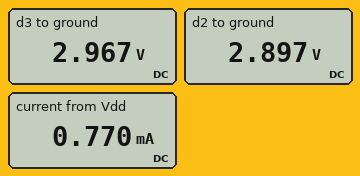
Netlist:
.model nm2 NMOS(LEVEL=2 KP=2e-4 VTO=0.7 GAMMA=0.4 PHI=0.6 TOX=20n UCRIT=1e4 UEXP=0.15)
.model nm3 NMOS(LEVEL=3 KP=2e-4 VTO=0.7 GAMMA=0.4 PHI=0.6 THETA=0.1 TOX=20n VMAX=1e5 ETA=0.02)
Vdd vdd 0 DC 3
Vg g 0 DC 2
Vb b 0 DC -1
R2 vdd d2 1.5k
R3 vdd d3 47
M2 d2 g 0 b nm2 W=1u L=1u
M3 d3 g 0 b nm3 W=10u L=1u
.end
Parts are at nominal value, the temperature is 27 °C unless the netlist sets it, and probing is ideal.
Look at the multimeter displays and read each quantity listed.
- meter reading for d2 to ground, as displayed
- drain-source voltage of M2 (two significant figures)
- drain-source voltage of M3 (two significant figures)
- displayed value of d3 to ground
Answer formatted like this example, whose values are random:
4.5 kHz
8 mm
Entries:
2.897 V
2.9 V
3.0 V
2.967 V
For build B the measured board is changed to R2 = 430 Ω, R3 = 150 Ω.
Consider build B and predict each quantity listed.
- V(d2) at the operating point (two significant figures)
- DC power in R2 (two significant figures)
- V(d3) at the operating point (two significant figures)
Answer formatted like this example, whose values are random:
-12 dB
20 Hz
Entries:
3.0 V
2.0 µW
2.9 V
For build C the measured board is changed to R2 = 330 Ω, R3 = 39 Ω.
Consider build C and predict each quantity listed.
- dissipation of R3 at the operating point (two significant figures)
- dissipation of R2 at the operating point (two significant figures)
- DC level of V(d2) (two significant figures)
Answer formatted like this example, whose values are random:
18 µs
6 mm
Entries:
19 µW
1.6 µW
3.0 V
